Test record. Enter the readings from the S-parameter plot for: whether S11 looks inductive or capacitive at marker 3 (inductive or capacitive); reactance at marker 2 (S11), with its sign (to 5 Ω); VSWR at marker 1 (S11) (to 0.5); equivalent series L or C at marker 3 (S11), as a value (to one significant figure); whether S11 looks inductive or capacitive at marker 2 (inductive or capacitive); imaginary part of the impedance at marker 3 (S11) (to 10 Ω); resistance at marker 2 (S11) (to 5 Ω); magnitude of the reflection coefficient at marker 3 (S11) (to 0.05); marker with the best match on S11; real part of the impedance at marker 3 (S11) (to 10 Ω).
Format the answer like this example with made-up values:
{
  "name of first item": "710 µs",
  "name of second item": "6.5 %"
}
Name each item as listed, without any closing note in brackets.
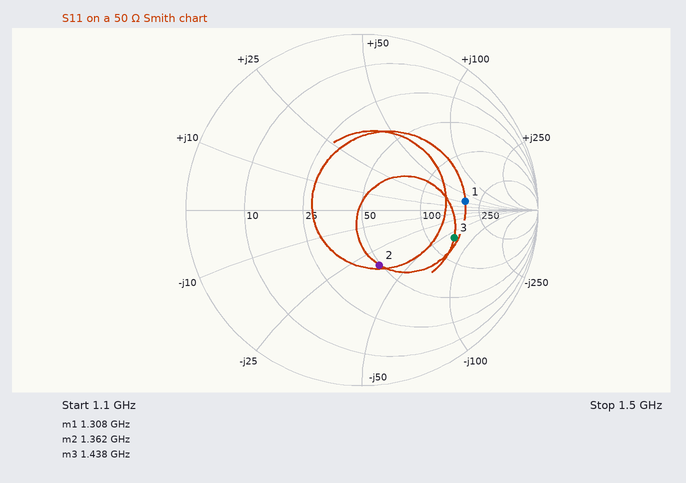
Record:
{
  "whether S11 looks inductive or capacitive at marker 3": "capacitive",
  "reactance at marker 2 (S11), with its sign": "-35 Ω",
  "VSWR at marker 1 (S11)": "4.0",
  "equivalent series L or C at marker 3 (S11), as a value": "2 pF",
  "whether S11 looks inductive or capacitive at marker 2": "capacitive",
  "imaginary part of the impedance at marker 3 (S11)": "-60 Ω",
  "resistance at marker 2 (S11)": "50 Ω",
  "magnitude of the reflection coefficient at marker 3 (S11)": "0.55",
  "marker with the best match on S11": "marker 2",
  "real part of the impedance at marker 3 (S11)": "140 Ω"
}
